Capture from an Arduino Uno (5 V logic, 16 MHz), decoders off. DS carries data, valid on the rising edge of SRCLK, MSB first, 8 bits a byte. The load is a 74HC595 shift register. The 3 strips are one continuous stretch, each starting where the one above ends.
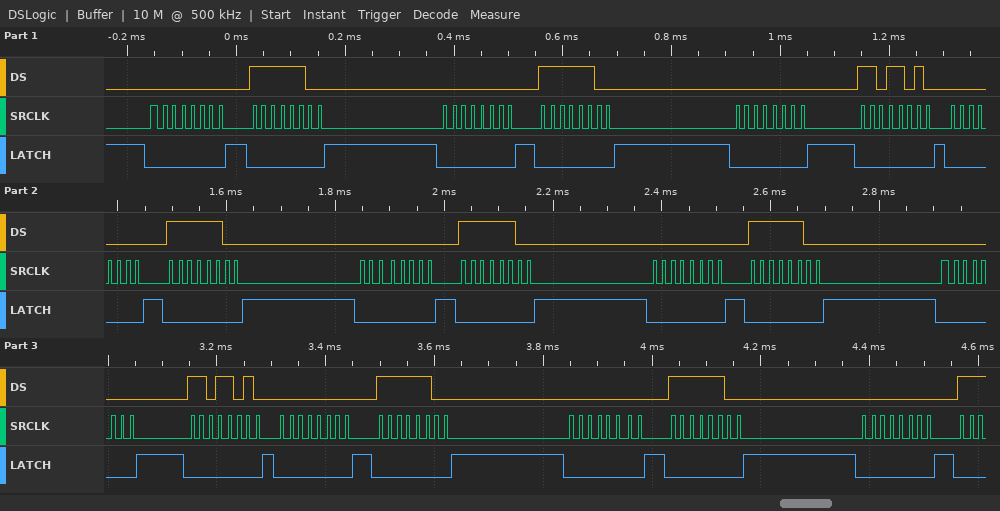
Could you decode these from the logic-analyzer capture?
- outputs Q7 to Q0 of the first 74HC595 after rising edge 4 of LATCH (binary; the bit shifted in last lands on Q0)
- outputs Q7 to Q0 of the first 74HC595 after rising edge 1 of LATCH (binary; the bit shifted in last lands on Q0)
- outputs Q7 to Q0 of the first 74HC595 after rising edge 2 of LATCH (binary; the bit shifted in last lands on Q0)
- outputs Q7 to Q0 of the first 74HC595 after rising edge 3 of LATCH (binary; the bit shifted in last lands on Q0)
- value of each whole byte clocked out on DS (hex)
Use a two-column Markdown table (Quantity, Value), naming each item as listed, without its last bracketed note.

| Quantity | Value |
|---|---|
| outputs Q7 to Q0 of the first 74HC595 after rising edge 4 of LATCH | 11111100 |
| outputs Q7 to Q0 of the first 74HC595 after rising edge 1 of LATCH | 00000000 |
| outputs Q7 to Q0 of the first 74HC595 after rising edge 2 of LATCH | 11111100 |
| outputs Q7 to Q0 of the first 74HC595 after rising edge 3 of LATCH | 00000000 |
| value of each whole byte clocked out on DS | 00 FC 00 FC 00 DA 00 FC 00 FC 00 FC 00 DA 00 FC 00 FC 00 |
